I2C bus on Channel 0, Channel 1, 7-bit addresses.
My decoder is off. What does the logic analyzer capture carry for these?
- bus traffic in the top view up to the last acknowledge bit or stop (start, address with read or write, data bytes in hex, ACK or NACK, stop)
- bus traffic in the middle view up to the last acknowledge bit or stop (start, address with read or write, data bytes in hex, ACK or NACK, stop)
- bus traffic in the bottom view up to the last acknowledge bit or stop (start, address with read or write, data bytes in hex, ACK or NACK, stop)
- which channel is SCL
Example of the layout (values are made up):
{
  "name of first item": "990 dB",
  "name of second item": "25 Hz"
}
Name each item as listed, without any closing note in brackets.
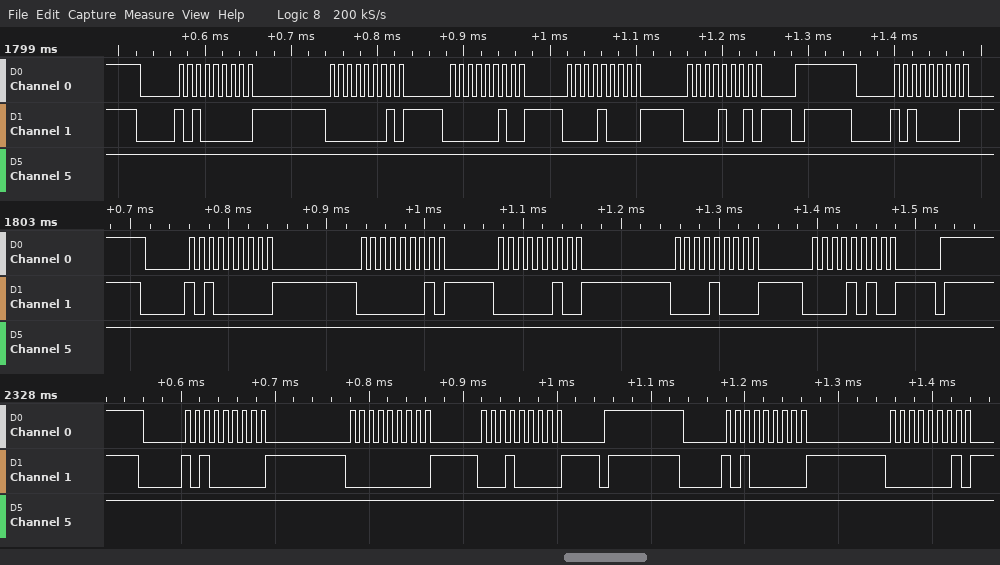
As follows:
{
  "bus traffic in the top view up to the last acknowledge bit or stop": "start, address 50 write ACK, 01 ACK, 02 ACK, 08 ACK, 09 ACK, stop, start, address 50 write NACK",
  "bus traffic in the middle view up to the last acknowledge bit or stop": "start, address 50 write ACK, 01 ACK, 02 ACK, 08 ACK, 0A ACK, stop",
  "bus traffic in the bottom view up to the last acknowledge bit or stop": "start, address 50 write ACK, 00 ACK, 10 ACK, stop, start, address 50 write ACK, 01 ACK",
  "which channel is SCL": "Channel 0"
}
